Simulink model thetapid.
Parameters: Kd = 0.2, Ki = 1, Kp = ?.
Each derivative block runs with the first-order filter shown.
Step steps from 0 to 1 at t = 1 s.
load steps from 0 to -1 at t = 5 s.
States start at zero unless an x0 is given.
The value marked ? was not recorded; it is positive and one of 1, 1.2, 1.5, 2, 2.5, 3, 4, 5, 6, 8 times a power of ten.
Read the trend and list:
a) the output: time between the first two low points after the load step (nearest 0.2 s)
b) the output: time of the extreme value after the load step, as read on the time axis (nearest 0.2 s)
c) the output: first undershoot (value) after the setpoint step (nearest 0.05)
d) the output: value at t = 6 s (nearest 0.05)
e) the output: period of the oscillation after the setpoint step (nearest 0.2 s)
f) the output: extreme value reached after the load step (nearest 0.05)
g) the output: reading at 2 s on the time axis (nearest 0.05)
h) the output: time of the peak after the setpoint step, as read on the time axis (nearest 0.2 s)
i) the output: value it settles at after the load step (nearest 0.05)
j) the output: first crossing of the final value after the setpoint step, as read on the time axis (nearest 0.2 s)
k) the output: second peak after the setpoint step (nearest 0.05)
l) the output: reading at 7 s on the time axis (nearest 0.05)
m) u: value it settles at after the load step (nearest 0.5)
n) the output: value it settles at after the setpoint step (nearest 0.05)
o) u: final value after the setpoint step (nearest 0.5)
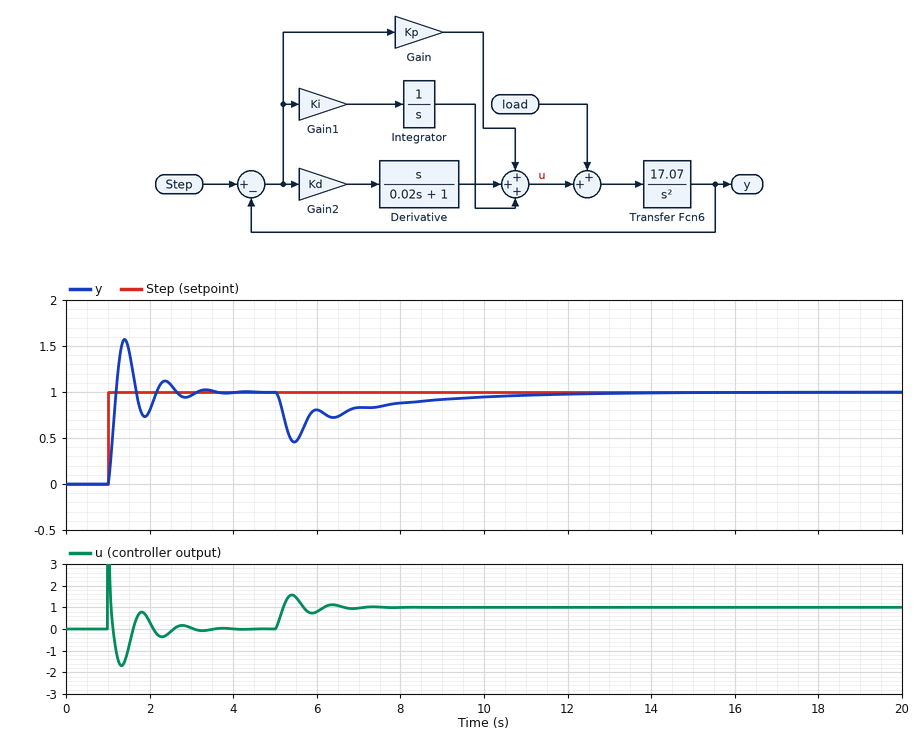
1.0 s
5.4 s
0.75
0.80
1.0 s
0.45
0.80
1.4 s
1.00
1.2 s
1.10
0.85
1.0
1.00
0.0
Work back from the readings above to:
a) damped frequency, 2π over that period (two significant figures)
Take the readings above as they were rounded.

6.3 rad/s
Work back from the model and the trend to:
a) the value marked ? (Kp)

2.5
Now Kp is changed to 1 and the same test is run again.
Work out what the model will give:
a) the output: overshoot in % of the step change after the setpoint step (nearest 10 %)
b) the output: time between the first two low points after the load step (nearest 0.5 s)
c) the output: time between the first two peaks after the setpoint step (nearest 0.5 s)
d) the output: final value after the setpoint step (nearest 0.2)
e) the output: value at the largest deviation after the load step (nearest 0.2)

50 %
1.5 s
1.5 s
1.0
0.0
